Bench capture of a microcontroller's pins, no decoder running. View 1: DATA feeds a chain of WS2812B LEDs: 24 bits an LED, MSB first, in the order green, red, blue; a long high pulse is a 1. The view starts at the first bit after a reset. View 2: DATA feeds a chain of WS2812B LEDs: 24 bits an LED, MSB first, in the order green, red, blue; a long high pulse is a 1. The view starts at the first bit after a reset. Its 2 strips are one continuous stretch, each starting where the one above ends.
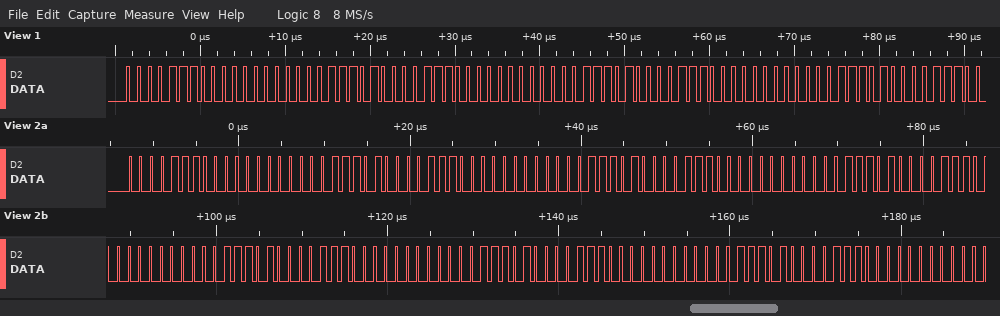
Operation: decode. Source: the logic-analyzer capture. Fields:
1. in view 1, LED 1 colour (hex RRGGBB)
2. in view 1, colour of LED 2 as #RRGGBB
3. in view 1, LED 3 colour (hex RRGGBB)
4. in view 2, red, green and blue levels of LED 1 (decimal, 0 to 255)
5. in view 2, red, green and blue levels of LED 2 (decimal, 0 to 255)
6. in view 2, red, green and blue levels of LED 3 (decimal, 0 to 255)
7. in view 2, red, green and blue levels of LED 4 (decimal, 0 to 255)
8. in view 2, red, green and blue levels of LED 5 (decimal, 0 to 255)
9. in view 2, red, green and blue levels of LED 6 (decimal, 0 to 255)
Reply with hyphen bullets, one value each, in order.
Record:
- #000E1D
- #000E1D
- #000E1D
- 0, 14, 29
- 0, 14, 29
- 0, 14, 29
- 0, 14, 29
- 0, 14, 29
- 0, 14, 29
